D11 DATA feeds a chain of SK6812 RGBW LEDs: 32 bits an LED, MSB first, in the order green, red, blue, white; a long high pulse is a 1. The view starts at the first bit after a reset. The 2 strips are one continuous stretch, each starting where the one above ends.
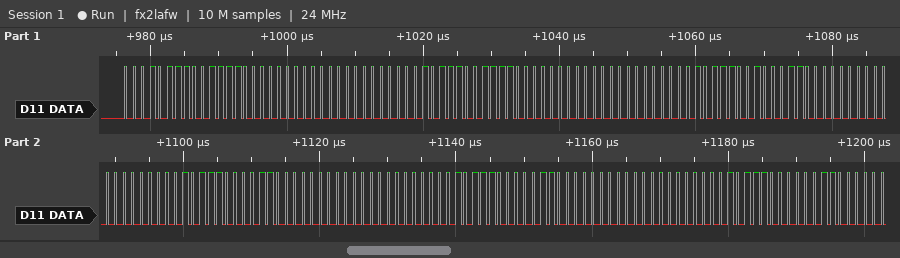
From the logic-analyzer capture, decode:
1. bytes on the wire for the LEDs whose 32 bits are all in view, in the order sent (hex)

17 3C 00 00 17 3C 00 00 17 23 00 00 17 0C 00 00 17 06 00 00
